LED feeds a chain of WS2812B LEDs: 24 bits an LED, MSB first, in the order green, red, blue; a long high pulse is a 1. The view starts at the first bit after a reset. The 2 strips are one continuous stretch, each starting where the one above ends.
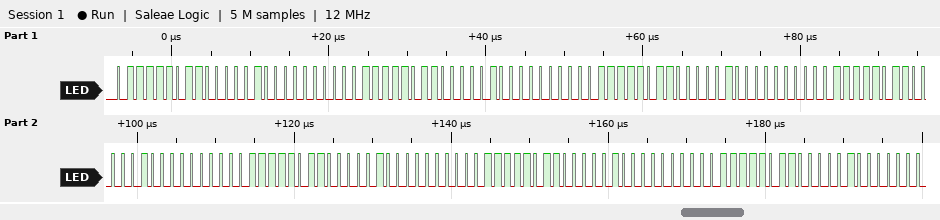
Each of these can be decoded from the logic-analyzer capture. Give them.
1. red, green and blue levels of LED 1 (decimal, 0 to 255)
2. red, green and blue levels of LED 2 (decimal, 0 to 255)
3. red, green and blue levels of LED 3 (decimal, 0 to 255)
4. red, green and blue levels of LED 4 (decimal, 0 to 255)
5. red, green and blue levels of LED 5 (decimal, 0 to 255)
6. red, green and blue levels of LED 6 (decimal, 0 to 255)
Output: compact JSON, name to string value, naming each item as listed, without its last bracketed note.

{"red, green and blue levels of LED 1": "130, 125, 0", "red, green and blue levels of LED 2": "130, 125, 0", "red, green and blue levels of LED 3": "130, 125, 0", "red, green and blue levels of LED 4": "130, 125, 0", "red, green and blue levels of LED 5": "130, 125, 0", "red, green and blue levels of LED 6": "130, 125, 0"}
